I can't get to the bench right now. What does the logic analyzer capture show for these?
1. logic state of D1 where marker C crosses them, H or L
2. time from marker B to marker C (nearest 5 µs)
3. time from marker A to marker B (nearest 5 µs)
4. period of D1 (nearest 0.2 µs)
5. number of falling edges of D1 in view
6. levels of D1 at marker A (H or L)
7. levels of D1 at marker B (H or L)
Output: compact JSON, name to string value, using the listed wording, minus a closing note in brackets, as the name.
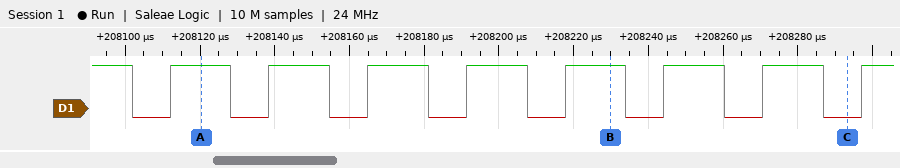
{"logic state of D1 where marker C crosses them, H or L": "D1=L", "time from marker B to marker C": "65 µs", "time from marker A to marker B": "110 µs", "period of D1": "26.4 µs", "number of falling edges of D1 in view": "8", "levels of D1 at marker A": "D1=H", "levels of D1 at marker B": "D1=H"}
